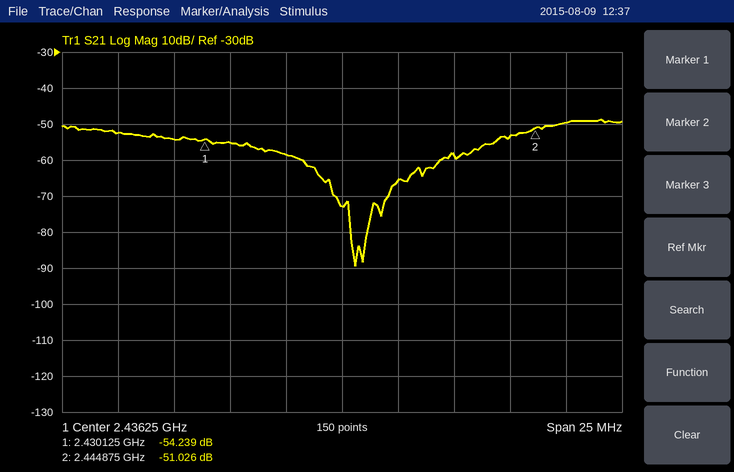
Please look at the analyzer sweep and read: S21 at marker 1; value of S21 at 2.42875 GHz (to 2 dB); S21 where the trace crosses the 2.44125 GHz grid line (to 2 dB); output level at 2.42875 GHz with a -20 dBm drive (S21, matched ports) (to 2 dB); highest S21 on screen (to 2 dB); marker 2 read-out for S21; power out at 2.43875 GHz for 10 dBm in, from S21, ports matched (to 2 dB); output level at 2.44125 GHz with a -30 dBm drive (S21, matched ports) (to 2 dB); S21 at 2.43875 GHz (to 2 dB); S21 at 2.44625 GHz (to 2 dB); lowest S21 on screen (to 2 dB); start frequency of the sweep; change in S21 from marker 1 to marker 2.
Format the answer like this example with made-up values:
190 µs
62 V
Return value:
-54.239 dB
-54 dB
-58 dB
-74 dBm
-48 dB
-51.026 dB
-56 dBm
-88 dBm
-66 dB
-50 dB
-90 dB
2.42375 GHz
3.213 dB
